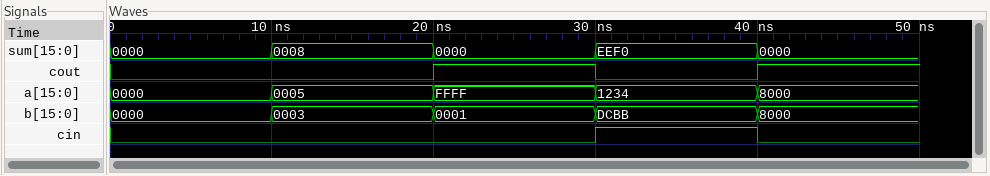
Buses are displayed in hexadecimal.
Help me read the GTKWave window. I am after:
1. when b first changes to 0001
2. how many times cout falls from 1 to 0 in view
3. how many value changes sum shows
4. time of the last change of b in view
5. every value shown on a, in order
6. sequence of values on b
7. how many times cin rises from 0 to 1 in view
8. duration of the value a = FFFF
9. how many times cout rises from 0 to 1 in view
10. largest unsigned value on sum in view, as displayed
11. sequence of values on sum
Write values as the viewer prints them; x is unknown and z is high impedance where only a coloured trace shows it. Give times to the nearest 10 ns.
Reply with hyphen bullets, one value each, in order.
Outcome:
- 20 ns
- 1
- 4
- 40 ns
- 0000, 0005, FFFF, 1234, 8000
- 0000, 0003, 0001, DCBB, 8000
- 1
- 10 ns
- 2
- EEF0
- 0000, 0008, 0000, EEF0, 0000
